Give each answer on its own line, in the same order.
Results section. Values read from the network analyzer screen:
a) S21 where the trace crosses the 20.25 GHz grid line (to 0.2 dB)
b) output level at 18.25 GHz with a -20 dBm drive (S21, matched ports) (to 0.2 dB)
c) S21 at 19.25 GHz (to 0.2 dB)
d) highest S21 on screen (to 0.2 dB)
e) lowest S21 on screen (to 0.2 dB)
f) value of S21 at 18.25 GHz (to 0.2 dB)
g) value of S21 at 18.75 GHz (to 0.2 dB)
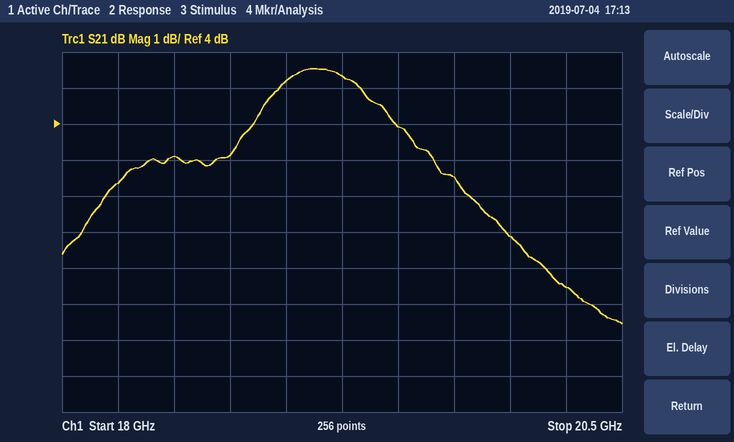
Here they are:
-0.6 dB
-17.6 dBm
5.4 dB
5.6 dB
-1.6 dB
2.4 dB
3.2 dB
